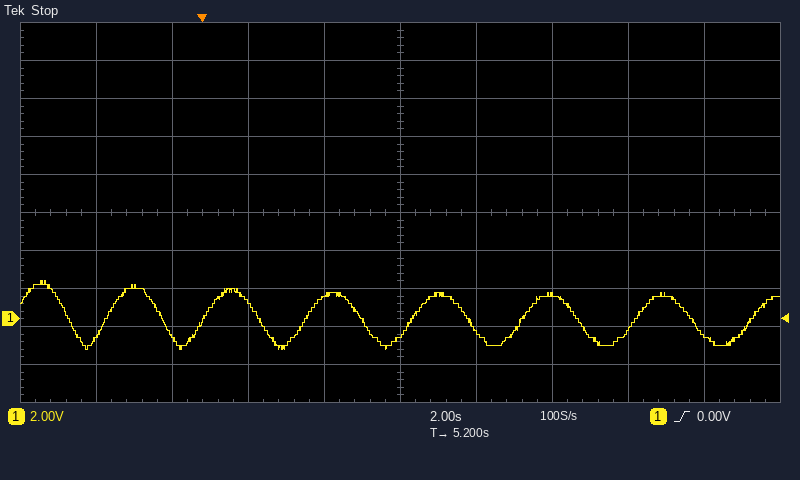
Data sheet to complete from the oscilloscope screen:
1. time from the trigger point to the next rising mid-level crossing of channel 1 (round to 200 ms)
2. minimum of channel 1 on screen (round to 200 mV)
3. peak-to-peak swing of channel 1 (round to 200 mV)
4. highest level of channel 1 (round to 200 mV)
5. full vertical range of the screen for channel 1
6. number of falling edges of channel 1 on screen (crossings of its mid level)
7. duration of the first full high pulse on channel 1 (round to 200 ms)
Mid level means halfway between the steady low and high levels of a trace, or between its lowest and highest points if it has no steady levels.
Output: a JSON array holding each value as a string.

["2.8 s", "-1.6 V", "3.6 V", "2.0 V", "20 V", "7", "1.4 s"]
